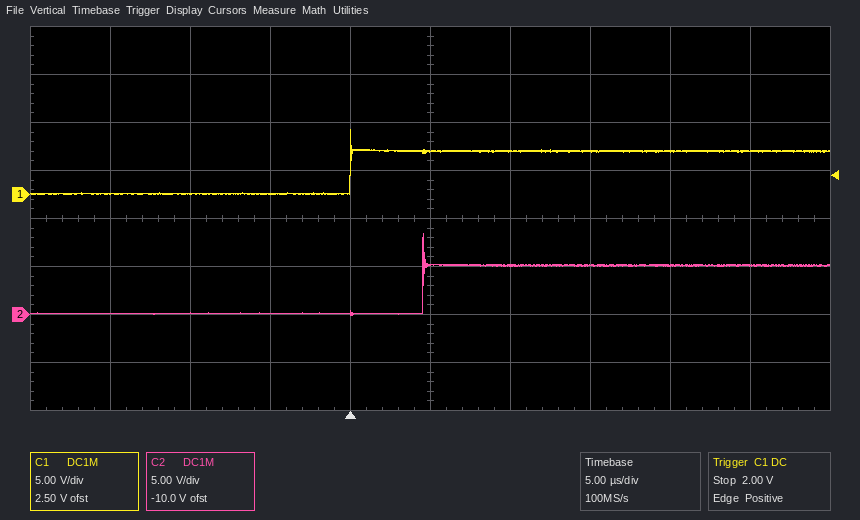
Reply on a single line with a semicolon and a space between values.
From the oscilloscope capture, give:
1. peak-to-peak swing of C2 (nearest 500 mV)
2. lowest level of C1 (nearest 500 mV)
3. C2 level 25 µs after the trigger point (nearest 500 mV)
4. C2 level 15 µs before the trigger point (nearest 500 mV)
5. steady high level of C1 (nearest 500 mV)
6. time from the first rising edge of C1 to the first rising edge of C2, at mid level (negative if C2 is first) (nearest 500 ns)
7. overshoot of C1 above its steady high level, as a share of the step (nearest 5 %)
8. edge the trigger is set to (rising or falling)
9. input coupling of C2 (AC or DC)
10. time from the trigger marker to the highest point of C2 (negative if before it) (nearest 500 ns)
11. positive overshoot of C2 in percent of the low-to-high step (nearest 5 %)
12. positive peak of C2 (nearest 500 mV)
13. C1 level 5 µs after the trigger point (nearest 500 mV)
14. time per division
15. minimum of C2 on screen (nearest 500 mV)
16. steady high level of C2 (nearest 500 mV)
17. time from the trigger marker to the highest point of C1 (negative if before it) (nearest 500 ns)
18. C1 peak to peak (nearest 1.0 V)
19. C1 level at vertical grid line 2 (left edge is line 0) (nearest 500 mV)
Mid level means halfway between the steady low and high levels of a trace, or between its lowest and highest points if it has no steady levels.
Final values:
8.5 V; 0.0 V; 5.0 V; 0.0 V; 4.5 V; +4.5 µs; 50 %; rising; DC; +4.5 µs; 65 %; 8.5 V; 4.5 V; 5 µs; 0.0 V; 5.0 V; 0.0 µs; 7.0 V; 0.0 V
